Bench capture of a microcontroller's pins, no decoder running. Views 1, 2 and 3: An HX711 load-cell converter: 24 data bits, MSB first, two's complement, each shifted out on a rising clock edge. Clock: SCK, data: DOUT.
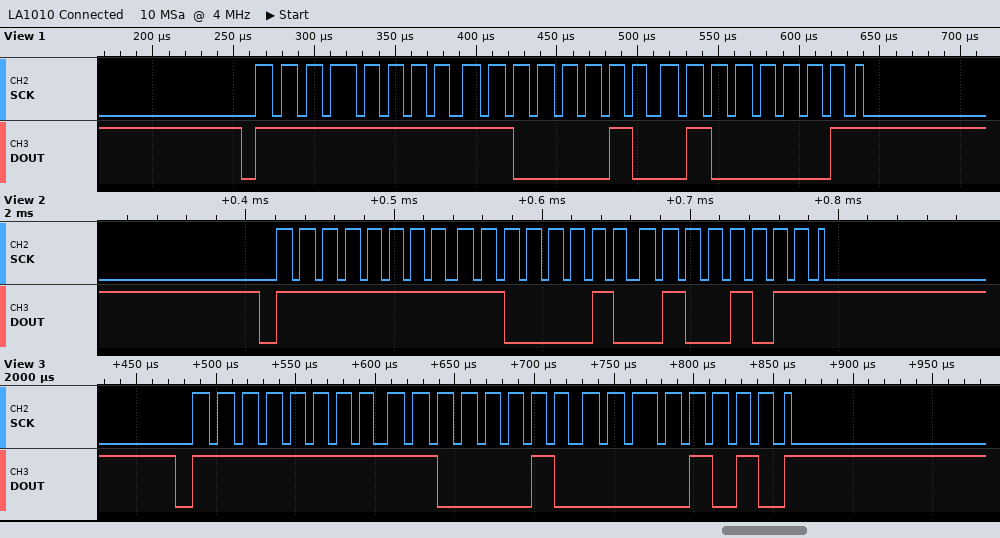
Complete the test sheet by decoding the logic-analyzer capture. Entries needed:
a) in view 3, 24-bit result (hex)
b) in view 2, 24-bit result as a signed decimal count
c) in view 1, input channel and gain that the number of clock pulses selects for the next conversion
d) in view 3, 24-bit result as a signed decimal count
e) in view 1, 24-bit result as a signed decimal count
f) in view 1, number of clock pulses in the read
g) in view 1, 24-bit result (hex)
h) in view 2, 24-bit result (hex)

0xFFC20A
-15797
channel A, gain 128
-15862
-15807
25
0xFFC241
0xFFC24B
